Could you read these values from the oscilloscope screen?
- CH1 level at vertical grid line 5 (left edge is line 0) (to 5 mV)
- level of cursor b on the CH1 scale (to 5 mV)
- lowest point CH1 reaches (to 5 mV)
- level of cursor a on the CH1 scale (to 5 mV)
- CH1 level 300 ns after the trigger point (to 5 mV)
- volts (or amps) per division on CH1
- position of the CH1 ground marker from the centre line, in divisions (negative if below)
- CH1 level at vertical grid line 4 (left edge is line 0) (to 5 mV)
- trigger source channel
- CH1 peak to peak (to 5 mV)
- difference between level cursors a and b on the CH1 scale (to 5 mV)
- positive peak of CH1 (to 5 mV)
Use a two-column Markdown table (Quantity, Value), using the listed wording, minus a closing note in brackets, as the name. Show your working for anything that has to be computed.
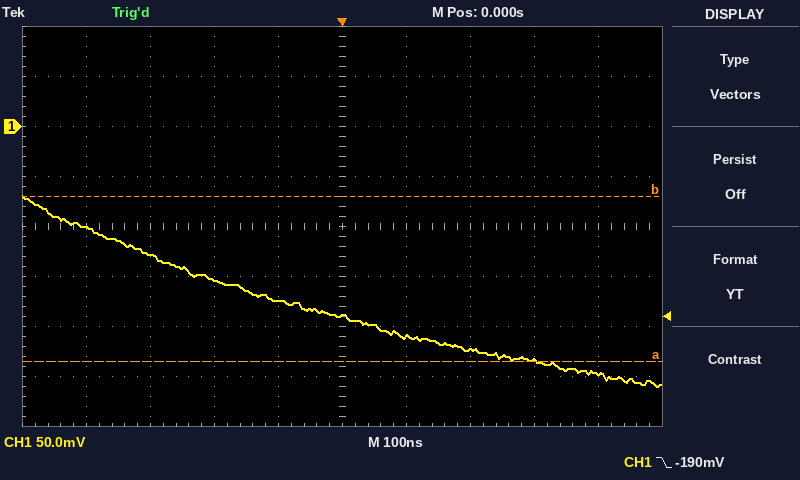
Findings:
| Quantity | Value |
|---|---|
| CH1 level at vertical grid line 5 (left edge is line 0) | -190 mV |
| level of cursor b on the CH1 scale | -70 mV |
| lowest point CH1 reaches | -260 mV |
| level of cursor a on the CH1 scale | -235 mV |
| CH1 level 300 ns after the trigger point | -235 mV |
| volts (or amps) per division on CH1 | 50 mV |
| position of the CH1 ground marker from the centre line, in divisions | +2.0 div |
| CH1 level at vertical grid line 4 (left edge is line 0) | -175 mV |
| trigger source channel | CH1 |
| CH1 peak to peak | -70 mV − (-260 mV) = 190 mV |
| difference between level cursors a and b on the CH1 scale | 165 mV |
| positive peak of CH1 | -70 mV |
